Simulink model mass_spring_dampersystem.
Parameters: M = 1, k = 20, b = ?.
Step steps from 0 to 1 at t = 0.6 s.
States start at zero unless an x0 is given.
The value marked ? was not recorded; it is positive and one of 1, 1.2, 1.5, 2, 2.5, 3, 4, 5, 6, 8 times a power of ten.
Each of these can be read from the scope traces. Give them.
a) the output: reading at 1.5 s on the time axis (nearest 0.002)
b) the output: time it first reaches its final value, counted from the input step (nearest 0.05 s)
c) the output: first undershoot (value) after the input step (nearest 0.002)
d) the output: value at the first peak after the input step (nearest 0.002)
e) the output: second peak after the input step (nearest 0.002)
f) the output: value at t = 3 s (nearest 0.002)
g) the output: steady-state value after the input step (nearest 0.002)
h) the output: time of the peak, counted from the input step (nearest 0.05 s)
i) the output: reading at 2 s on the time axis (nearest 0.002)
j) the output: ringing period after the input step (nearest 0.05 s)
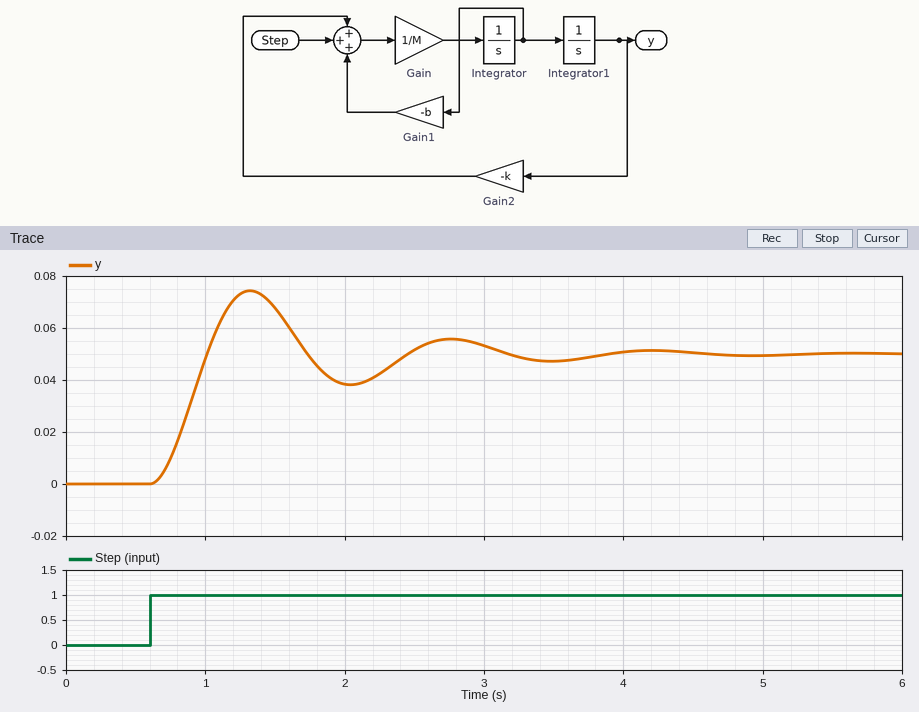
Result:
0.068
0.40 s
0.038
0.074
0.056
0.054
0.050
0.70 s
0.038
1.45 s
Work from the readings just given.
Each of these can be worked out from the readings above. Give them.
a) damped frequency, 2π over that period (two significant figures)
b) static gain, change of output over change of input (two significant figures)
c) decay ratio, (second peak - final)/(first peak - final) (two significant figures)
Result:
4.3 rad/s
0.050
0.25
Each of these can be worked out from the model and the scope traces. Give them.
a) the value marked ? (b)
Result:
2
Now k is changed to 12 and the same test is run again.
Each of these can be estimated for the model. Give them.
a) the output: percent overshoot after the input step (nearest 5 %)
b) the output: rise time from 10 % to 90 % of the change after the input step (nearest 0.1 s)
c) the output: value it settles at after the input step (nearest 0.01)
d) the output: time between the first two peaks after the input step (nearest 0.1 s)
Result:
40 %
0.4 s
0.08
1.9 s
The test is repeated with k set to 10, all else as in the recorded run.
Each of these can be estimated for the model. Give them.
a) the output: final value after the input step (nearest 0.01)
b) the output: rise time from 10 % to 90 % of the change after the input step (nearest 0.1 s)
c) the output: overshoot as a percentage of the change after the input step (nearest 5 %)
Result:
0.10
0.4 s
35 %
